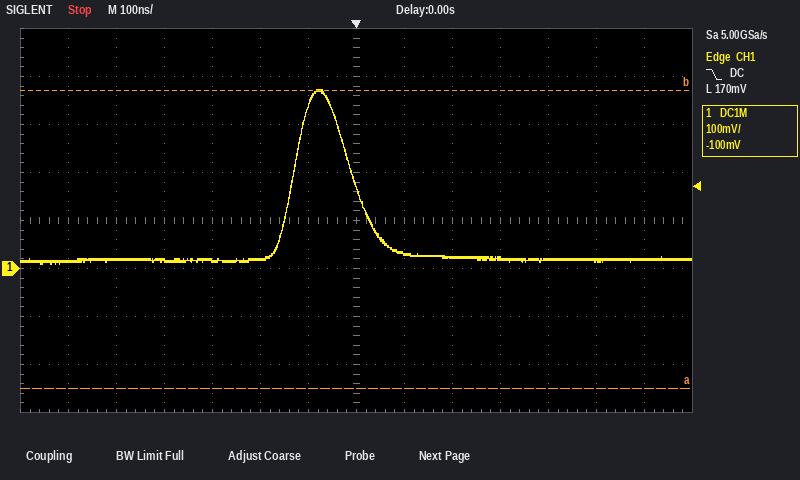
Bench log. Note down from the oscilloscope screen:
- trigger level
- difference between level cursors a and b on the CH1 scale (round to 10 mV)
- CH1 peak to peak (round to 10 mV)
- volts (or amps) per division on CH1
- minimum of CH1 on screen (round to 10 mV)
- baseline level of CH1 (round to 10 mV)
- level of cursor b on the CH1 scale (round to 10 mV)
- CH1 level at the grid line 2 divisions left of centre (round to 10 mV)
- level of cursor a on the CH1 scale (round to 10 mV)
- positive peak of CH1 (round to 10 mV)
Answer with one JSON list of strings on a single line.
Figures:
["170 mV", "620 mV", "360 mV", "100 mV", "10 mV", "20 mV", "370 mV", "20 mV", "-250 mV", "370 mV"]
